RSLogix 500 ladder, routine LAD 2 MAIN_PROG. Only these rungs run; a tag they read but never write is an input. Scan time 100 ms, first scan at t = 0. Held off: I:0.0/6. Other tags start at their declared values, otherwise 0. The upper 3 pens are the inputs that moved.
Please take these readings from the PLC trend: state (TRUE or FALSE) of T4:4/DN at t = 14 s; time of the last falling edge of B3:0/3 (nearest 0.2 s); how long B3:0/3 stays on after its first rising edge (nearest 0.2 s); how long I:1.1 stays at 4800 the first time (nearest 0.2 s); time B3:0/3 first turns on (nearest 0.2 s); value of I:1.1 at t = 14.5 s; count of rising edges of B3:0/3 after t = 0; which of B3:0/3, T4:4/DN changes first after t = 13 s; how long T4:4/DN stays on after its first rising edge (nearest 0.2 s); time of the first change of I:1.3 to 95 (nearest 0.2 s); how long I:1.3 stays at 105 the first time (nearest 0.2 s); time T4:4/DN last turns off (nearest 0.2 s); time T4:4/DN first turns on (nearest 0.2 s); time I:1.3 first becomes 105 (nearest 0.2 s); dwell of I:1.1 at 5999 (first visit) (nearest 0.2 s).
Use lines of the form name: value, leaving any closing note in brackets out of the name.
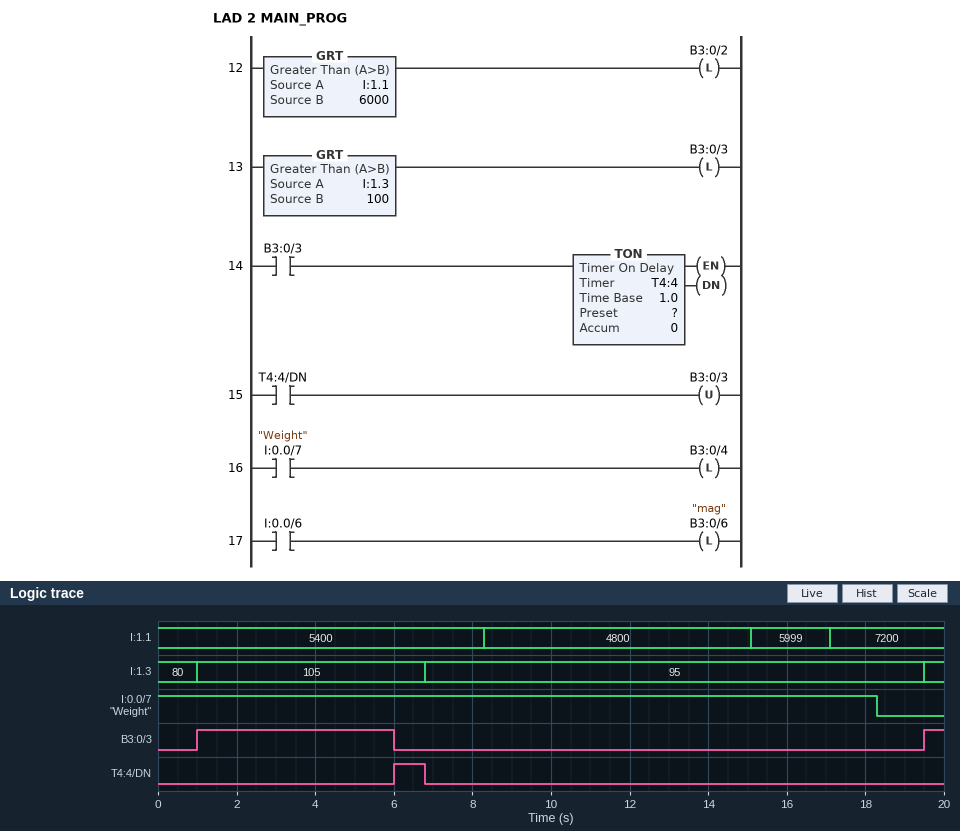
state (TRUE or FALSE) of T4:4/DN at t = 14 s: FALSE
time of the last falling edge of B3:0/3: 6.0 s
how long B3:0/3 stays on after its first rising edge: 5.0 s
how long I:1.1 stays at 4800 the first time: 6.8 s
time B3:0/3 first turns on: 1.0 s
value of I:1.1 at t = 14.5 s: 4800
count of rising edges of B3:0/3 after t = 0: 2
which of B3:0/3, T4:4/DN changes first after t = 13 s: B3:0/3
how long T4:4/DN stays on after its first rising edge: 0.8 s
time of the first change of I:1.3 to 95: 6.8 s
how long I:1.3 stays at 105 the first time: 5.8 s
time T4:4/DN last turns off: 6.8 s
time T4:4/DN first turns on: 6.0 s
time I:1.3 first becomes 105: 1.0 s
dwell of I:1.1 at 5999 (first visit): 2.0 s
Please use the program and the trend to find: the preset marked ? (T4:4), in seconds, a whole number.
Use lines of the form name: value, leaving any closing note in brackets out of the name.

the preset marked ? (T4:4), in seconds, a whole number: 5 s
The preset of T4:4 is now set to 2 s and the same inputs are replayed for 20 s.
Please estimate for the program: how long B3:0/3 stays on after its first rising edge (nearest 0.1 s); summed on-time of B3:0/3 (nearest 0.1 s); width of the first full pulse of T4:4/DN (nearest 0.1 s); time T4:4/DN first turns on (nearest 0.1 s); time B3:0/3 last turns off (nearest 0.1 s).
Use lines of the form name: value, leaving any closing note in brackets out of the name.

how long B3:0/3 stays on after its first rising edge: 2.0 s
summed on-time of B3:0/3: 2.5 s
width of the first full pulse of T4:4/DN: 3.8 s
time T4:4/DN first turns on: 3.0 s
time B3:0/3 last turns off: 3.0 s
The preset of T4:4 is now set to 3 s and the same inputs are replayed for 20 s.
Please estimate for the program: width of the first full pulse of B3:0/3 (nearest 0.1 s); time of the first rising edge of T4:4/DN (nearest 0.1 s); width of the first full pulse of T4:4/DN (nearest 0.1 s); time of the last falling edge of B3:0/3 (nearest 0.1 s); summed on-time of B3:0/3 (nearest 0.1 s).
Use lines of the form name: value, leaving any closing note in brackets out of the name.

width of the first full pulse of B3:0/3: 3.0 s
time of the first rising edge of T4:4/DN: 4.0 s
width of the first full pulse of T4:4/DN: 2.8 s
time of the last falling edge of B3:0/3: 4.0 s
summed on-time of B3:0/3: 3.5 s
